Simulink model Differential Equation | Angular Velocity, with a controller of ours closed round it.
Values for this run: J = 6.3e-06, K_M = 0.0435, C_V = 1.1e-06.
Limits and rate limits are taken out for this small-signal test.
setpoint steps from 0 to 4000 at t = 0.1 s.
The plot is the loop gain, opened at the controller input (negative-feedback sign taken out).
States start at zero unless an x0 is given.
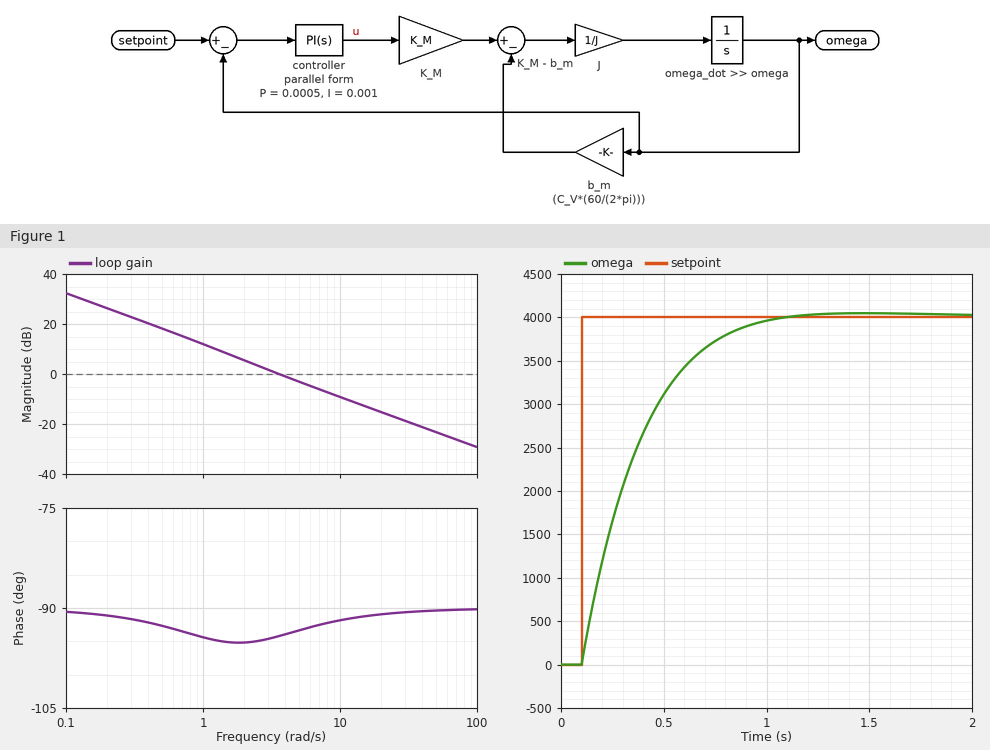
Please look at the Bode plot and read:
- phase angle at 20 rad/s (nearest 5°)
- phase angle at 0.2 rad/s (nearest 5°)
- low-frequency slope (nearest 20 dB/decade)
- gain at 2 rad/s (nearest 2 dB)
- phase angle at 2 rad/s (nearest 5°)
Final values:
-90°
-90°
-20 dB/decade
6 dB
-95°
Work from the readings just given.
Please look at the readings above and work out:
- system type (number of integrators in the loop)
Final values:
1
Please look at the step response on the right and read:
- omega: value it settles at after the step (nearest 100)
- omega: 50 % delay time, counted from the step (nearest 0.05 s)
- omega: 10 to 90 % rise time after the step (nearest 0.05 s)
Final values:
4000
0.20 s
0.55 s
